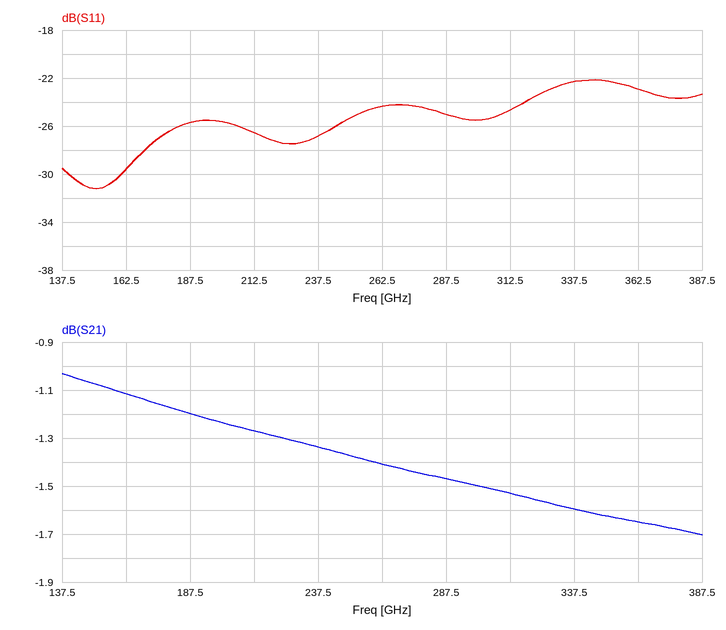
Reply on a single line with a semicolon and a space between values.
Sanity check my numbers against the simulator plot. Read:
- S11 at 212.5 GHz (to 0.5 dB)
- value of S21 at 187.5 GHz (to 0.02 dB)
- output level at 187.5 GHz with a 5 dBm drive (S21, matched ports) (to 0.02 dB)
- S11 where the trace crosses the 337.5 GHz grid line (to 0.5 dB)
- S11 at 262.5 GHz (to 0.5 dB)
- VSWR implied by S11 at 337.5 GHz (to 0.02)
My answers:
-26.5 dB; -1.20 dB; 3.80 dBm; -22.5 dB; -24.5 dB; 1.16
